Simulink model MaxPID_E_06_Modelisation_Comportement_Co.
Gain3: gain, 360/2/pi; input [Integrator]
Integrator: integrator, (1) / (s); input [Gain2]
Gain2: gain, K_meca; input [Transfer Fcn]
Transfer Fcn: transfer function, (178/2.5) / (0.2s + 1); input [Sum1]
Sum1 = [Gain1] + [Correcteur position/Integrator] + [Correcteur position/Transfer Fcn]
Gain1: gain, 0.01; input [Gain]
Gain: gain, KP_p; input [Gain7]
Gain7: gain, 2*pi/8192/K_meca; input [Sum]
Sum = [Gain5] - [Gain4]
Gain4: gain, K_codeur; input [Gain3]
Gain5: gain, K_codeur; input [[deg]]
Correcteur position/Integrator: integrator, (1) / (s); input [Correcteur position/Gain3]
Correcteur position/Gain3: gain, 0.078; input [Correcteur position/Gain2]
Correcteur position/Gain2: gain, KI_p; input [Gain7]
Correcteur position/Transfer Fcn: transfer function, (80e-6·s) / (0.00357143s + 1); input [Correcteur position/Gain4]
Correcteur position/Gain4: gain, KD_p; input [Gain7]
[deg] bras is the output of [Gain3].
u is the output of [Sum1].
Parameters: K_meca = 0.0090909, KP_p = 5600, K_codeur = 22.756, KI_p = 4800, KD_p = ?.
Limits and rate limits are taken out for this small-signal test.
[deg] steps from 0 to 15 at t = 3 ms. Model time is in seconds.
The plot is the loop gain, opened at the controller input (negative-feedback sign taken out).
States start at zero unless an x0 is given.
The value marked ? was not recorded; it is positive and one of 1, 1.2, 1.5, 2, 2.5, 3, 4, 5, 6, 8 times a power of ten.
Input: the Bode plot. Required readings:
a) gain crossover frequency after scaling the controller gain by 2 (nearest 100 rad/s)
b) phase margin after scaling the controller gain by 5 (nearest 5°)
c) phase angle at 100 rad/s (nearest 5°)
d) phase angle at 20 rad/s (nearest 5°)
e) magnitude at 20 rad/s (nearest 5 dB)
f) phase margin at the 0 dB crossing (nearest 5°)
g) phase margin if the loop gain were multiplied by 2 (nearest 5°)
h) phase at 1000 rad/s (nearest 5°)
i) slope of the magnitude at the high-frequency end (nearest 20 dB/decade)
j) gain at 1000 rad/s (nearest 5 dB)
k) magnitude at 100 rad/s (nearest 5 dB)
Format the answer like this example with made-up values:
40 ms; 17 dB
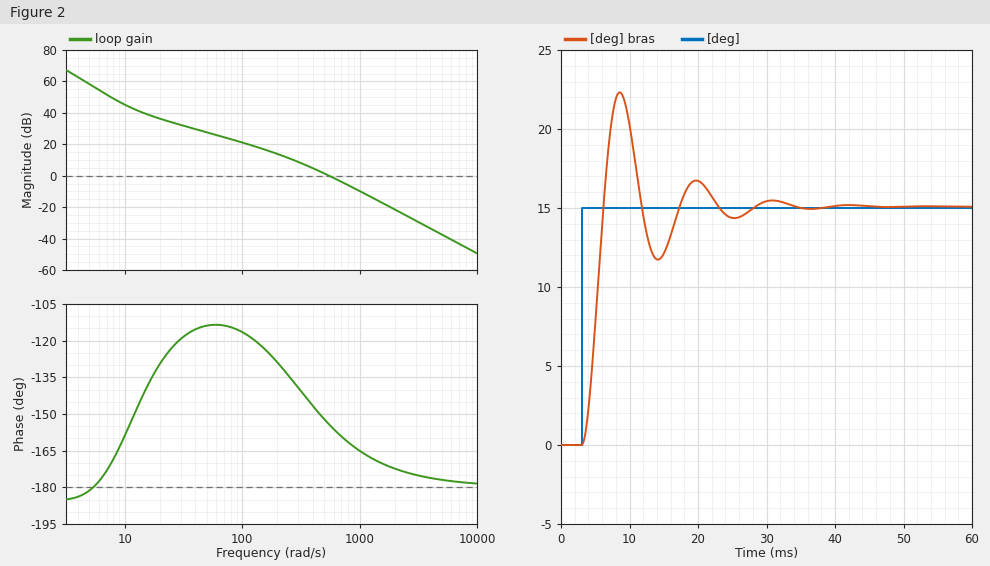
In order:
800 rad/s; 10°; -115°; -130°; 35 dB; 25°; 20°; -165°; -40 dB/decade; -10 dB; 20 dB
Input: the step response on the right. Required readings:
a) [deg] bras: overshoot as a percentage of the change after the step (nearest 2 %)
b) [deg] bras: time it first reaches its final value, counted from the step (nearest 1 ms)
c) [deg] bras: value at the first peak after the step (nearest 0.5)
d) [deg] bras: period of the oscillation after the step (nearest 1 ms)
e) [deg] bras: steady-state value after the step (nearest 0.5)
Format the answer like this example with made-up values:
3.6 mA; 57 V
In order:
48 %; 3 ms; 22.5; 11 ms; 15.0
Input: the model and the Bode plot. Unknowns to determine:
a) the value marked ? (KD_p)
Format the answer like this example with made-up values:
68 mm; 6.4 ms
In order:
40000
